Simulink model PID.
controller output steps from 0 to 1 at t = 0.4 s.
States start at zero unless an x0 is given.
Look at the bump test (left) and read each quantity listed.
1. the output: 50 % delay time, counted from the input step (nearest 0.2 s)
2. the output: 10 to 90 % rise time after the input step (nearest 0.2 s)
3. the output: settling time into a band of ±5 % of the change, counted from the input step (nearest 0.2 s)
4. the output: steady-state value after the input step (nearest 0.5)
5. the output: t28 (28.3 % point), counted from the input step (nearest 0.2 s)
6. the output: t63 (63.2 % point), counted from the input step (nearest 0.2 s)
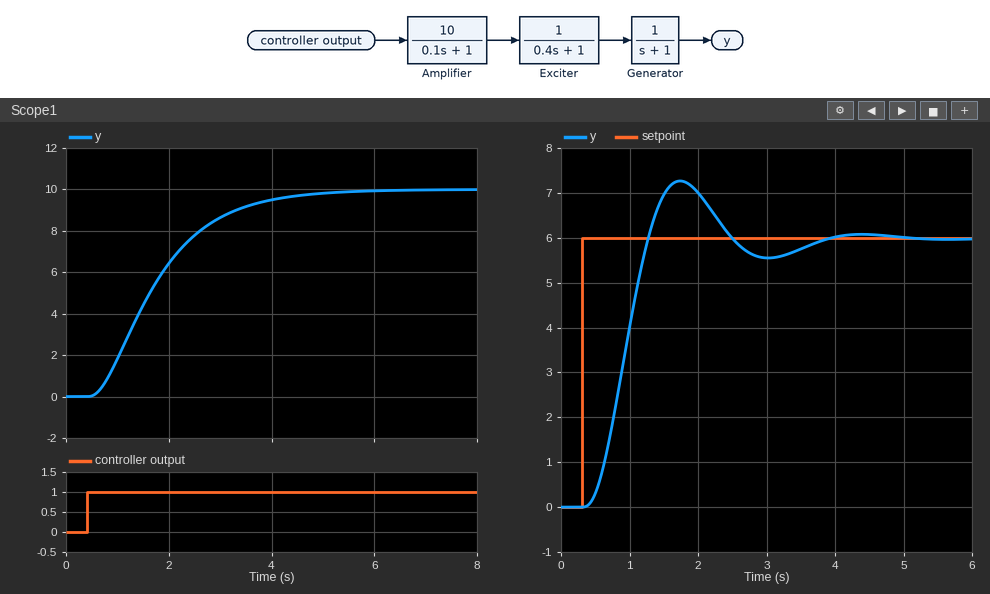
1.2 s
2.4 s
3.6 s
10.0
0.8 s
1.6 s
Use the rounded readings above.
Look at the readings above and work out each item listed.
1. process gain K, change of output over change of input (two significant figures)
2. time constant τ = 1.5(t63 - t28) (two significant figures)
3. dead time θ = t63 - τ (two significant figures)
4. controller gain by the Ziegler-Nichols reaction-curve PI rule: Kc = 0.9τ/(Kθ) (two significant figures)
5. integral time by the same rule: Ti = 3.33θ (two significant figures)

10
1.2 s
0.40 s
0.27
1.3 s
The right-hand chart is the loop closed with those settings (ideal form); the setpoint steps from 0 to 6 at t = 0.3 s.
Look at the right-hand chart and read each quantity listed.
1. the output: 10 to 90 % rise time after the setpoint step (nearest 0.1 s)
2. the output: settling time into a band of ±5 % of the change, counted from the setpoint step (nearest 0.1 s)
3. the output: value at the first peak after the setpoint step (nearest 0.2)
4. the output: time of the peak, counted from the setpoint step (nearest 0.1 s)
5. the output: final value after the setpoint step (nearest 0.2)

0.6 s
3.1 s
7.2
1.4 s
6.0
